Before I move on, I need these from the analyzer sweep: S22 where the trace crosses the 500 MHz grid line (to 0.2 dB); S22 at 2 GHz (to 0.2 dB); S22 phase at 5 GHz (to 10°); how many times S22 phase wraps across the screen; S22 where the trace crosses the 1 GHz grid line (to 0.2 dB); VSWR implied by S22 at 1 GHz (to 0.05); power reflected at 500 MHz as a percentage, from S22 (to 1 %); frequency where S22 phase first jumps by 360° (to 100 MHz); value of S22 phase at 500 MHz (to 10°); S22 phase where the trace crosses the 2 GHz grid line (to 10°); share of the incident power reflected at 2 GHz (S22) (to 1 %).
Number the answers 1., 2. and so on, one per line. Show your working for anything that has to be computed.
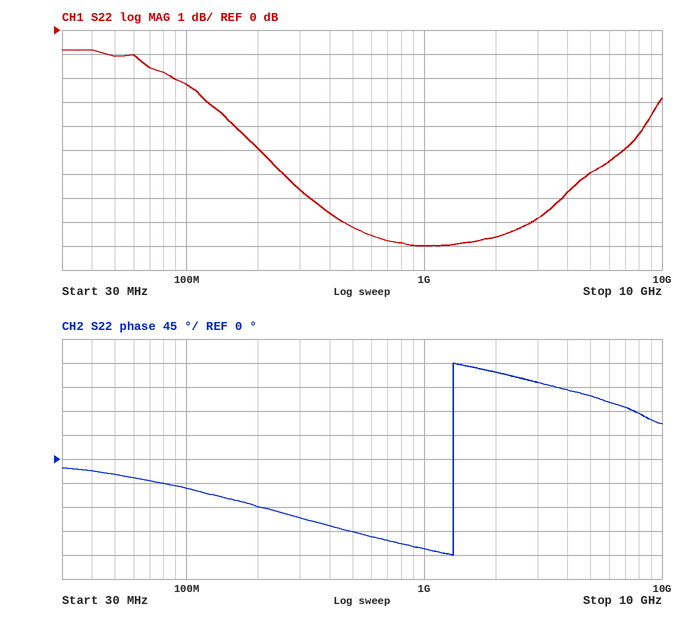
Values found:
1. -8.2 dB
2. -8.6 dB
3. 120°
4. 1
5. -9.0 dB
6. |Γ| = 10^(-9/20) = 0.3548; VSWR = (1 + 0.3548)/(1 − 0.3548) ≈ 2.10
7. 10^(-8.2/10) ≈ 15 %
8. 1.3 GHz
9. -140°
10. 160°
11. 10^(-8.6/10) ≈ 14 %
